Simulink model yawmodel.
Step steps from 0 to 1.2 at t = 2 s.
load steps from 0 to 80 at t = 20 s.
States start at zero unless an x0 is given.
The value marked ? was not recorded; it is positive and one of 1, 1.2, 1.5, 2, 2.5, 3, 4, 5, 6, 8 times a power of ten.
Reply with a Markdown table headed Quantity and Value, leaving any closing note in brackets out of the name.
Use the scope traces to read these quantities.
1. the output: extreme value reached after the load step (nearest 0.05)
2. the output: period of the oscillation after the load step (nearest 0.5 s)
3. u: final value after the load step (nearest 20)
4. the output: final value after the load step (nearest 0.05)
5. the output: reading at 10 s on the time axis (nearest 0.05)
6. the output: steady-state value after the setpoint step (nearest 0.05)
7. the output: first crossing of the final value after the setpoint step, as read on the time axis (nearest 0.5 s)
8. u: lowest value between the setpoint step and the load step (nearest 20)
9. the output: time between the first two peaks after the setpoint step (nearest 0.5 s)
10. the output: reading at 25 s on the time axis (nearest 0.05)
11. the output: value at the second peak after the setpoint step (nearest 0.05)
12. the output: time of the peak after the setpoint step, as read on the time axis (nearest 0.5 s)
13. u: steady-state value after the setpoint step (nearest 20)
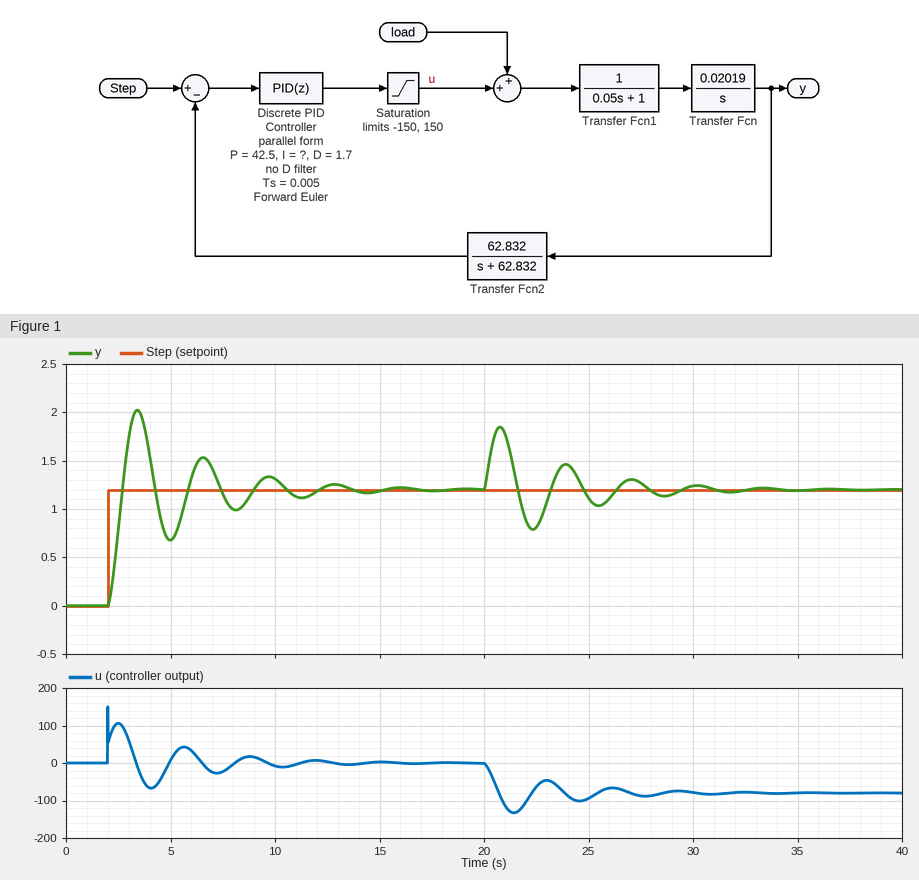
| Quantity | Value |
|---|---|
| the output: extreme value reached after the load step | 1.85 |
| the output: period of the oscillation after the load step | 3.0 s |
| u: final value after the load step | -80 |
| the output: final value after the load step | 1.20 |
| the output: reading at 10 s on the time axis | 1.30 |
| the output: steady-state value after the setpoint step | 1.20 |
| the output: first crossing of the final value after the setpoint step, as read on the time axis | 2.5 s |
| u: lowest value between the setpoint step and the load step | -60 |
| the output: time between the first two peaks after the setpoint step | 3.0 s |
| the output: reading at 25 s on the time axis | 1.10 |
| the output: value at the second peak after the setpoint step | 1.55 |
| the output: time of the peak after the setpoint step, as read on the time axis | 3.5 s |
| u: steady-state value after the setpoint step | 0 |
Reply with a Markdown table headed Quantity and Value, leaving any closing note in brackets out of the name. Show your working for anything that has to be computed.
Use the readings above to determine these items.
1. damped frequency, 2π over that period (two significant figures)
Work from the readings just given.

| Quantity | Value |
|---|---|
| damped frequency, 2π over that period | 2π / 3 = 2.1 rad/s |
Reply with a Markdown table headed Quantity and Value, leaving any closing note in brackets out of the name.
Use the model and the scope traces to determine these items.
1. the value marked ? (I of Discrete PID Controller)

| Quantity | Value |
|---|---|
| the value marked ? | 200 |
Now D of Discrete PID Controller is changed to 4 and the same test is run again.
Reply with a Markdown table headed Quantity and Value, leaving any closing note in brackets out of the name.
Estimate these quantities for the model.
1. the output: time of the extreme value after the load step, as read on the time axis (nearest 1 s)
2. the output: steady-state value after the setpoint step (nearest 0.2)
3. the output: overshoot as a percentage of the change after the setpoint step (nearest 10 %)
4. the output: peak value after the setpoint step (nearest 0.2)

| Quantity | Value |
|---|---|
| the output: time of the extreme value after the load step, as read on the time axis | 21 s |
| the output: steady-state value after the setpoint step | 1.2 |
| the output: overshoot as a percentage of the change after the setpoint step | 70 % |
| the output: peak value after the setpoint step | 2.0 |
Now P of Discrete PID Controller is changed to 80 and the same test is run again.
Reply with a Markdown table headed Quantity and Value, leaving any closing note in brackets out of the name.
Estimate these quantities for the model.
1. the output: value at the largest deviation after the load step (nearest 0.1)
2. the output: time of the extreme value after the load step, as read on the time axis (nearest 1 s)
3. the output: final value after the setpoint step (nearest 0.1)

| Quantity | Value |
|---|---|
| the output: value at the largest deviation after the load step | 1.7 |
| the output: time of the extreme value after the load step, as read on the time axis | 21 s |
| the output: final value after the setpoint step | 1.2 |
